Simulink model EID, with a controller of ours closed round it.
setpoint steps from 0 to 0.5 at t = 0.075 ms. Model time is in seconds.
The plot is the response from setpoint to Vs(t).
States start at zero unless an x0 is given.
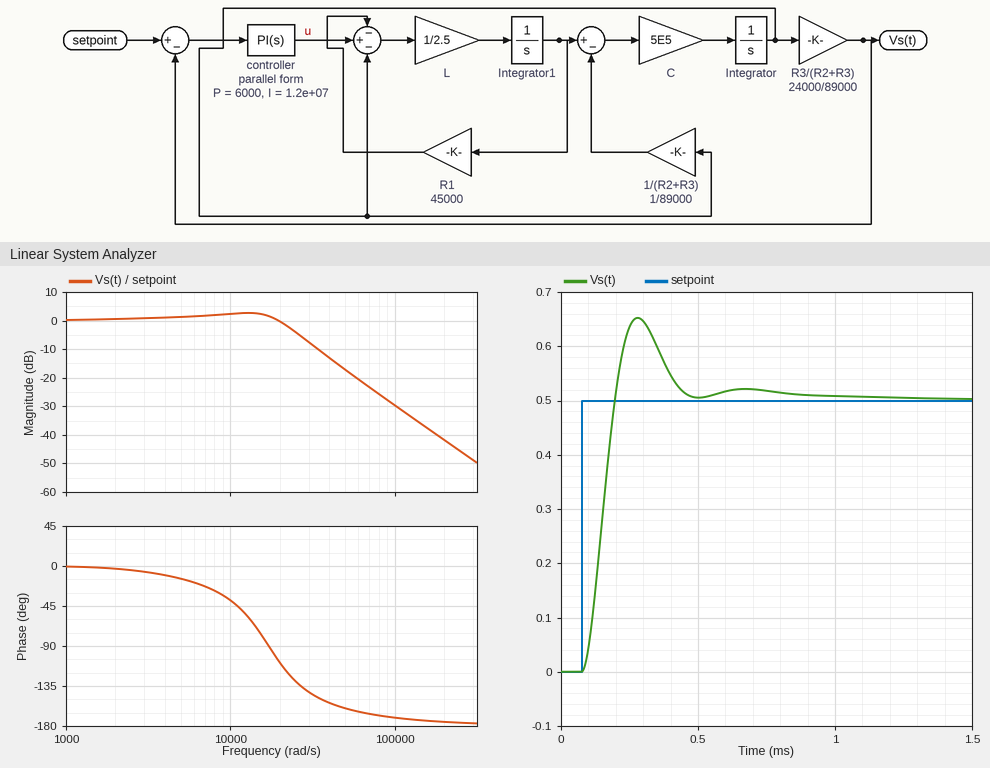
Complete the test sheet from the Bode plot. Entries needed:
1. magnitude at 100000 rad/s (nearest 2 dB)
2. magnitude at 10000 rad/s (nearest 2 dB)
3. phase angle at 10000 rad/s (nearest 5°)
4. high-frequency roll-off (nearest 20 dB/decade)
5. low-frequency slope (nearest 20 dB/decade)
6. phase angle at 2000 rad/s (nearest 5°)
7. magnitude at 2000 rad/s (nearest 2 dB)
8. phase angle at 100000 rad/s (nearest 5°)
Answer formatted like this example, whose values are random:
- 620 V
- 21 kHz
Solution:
- -30 dB
- 2 dB
- -40°
- -40 dB/decade
- 0 dB/decade
- -5°
- 0 dB
- -170°
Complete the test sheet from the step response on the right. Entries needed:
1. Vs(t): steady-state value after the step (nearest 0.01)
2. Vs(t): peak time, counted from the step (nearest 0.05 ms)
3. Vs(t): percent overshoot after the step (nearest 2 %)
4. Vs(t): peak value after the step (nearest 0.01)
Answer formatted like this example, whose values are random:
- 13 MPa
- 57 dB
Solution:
- 0.50
- 0.20 ms
- 30 %
- 0.65
